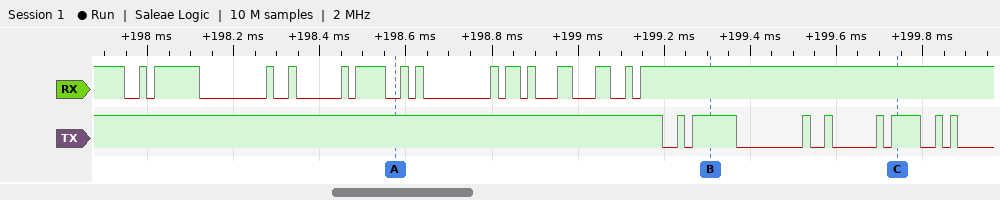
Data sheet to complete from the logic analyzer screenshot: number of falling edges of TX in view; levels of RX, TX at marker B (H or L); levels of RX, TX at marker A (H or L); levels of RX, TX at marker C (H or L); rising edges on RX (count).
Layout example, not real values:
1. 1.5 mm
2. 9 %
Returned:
1. 9
2. RX=H, TX=H
3. RX=L, TX=H
4. RX=H, TX=H
5. 15
